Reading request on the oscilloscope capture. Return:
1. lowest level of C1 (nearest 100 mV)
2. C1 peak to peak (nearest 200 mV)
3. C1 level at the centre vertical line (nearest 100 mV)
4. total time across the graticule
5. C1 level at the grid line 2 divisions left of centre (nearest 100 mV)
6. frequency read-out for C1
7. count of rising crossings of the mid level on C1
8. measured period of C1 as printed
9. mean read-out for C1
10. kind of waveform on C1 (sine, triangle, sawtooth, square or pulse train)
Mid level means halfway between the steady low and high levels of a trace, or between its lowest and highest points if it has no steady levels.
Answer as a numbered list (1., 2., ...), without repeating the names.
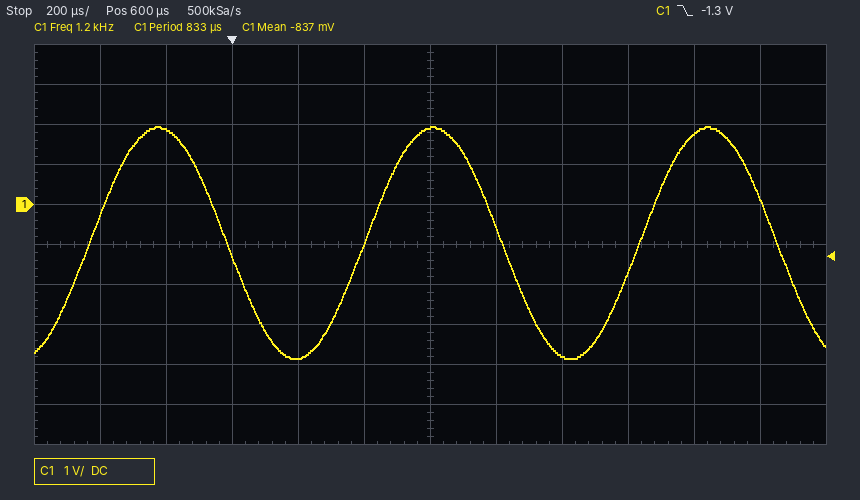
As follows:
1. -3.8 V
2. 5.8 V
3. 1.9 V
4. 2.4 ms
5. -3.8 V
6. 1.2 kHz
7. 3
8. 833 µs
9. -837 mV
10. sine
